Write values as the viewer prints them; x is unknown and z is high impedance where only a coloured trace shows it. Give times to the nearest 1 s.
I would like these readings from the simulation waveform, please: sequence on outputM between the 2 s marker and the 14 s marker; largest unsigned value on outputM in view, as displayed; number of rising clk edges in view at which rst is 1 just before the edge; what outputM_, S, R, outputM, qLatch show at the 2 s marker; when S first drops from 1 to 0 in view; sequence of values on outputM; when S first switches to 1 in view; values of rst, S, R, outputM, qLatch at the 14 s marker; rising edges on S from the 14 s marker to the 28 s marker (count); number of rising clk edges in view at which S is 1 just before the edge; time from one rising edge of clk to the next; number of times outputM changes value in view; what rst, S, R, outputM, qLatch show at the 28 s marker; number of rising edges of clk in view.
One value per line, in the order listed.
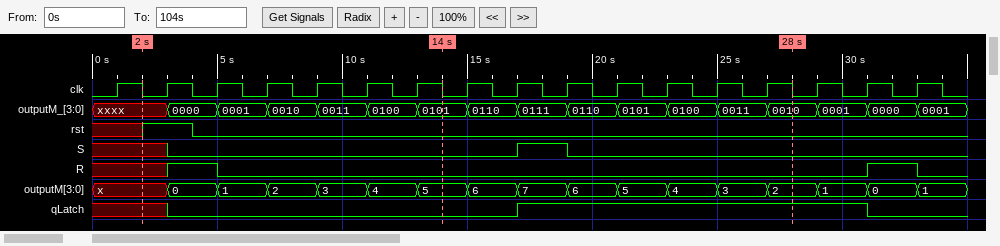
x, 0, 1, 2, 3, 4, 5
7
1
outputM_=xxxx, S=x, R=x, outputM=x, qLatch=x
19 s
x, 0, 1, 2, 3, 4, 5, 6, 7, 6, 5, 4, 3, 2, 1, 0, 1
17 s
rst=0, S=0, R=0, outputM=5, qLatch=0
1
1
2 s
16
rst=0, S=0, R=0, outputM=2, qLatch=1
17
